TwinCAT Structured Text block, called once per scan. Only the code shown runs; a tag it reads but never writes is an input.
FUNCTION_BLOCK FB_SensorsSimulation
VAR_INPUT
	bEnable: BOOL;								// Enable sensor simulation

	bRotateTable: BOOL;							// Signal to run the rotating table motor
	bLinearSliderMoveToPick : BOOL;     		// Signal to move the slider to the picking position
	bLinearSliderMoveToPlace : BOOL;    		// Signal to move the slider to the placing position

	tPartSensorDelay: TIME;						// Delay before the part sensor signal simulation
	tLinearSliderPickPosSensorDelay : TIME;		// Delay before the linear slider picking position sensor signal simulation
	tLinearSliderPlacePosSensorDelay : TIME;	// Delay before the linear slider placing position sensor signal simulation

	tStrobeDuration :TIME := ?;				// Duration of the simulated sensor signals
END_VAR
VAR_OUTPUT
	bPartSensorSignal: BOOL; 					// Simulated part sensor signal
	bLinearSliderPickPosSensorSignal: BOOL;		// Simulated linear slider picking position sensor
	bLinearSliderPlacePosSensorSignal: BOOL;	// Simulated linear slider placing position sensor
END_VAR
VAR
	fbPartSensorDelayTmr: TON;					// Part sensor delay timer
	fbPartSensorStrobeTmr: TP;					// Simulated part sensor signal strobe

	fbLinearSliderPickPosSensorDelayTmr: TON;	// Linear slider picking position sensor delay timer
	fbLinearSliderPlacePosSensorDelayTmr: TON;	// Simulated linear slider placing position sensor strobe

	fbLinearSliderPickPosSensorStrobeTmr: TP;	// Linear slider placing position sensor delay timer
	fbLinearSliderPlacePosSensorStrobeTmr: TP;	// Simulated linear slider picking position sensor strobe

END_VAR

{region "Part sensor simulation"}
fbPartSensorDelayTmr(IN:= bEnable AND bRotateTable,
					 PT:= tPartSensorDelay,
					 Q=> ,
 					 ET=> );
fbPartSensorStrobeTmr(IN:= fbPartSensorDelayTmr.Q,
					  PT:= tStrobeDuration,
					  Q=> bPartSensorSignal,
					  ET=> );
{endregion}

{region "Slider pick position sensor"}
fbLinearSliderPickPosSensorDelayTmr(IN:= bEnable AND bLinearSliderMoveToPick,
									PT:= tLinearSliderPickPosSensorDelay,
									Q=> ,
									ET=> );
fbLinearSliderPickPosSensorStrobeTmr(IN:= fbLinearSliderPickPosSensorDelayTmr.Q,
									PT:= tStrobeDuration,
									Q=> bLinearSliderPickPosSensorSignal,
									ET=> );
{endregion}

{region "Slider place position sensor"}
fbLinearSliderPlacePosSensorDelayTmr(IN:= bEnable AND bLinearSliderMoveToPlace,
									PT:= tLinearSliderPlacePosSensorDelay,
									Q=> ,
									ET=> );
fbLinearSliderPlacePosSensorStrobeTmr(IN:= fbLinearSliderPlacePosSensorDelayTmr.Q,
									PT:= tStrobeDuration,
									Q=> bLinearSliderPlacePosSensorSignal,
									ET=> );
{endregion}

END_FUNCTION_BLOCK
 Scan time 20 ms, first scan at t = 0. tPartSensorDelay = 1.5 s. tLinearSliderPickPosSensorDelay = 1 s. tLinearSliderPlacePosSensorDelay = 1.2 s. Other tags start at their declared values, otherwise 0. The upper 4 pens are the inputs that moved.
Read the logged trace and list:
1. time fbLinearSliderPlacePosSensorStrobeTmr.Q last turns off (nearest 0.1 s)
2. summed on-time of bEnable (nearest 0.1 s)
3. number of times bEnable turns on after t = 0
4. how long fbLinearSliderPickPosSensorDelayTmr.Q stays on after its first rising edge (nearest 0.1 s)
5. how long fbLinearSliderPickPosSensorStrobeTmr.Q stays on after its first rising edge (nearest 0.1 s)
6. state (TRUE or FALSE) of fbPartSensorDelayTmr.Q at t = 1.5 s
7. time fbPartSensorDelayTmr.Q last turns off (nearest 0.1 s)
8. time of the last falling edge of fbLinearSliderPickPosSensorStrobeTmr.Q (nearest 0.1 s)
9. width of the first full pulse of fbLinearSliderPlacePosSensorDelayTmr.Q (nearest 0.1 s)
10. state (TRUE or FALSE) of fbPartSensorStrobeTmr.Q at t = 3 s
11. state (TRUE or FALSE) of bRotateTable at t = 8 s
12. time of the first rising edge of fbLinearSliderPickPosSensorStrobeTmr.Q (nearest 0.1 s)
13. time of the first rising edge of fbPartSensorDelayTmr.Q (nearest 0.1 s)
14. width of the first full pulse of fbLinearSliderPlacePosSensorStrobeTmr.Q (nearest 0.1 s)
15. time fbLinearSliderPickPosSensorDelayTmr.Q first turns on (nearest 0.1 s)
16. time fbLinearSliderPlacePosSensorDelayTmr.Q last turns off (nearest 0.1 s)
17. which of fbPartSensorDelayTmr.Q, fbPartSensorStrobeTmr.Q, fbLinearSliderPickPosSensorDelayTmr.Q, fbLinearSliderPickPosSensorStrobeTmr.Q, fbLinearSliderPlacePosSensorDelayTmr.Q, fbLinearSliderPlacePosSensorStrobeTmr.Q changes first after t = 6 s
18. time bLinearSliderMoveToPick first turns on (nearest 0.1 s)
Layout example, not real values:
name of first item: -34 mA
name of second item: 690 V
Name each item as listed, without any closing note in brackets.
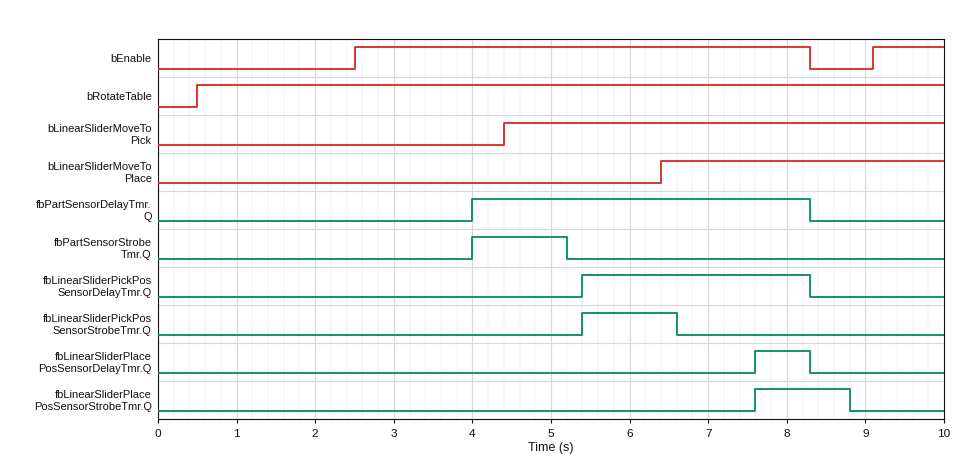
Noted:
time fbLinearSliderPlacePosSensorStrobeTmr.Q last turns off: 8.8 s
summed on-time of bEnable: 6.7 s
number of times bEnable turns on after t = 0: 2
how long fbLinearSliderPickPosSensorDelayTmr.Q stays on after its first rising edge: 2.9 s
how long fbLinearSliderPickPosSensorStrobeTmr.Q stays on after its first rising edge: 1.2 s
state (TRUE or FALSE) of fbPartSensorDelayTmr.Q at t = 1.5 s: FALSE
time fbPartSensorDelayTmr.Q last turns off: 8.3 s
time of the last falling edge of fbLinearSliderPickPosSensorStrobeTmr.Q: 6.6 s
width of the first full pulse of fbLinearSliderPlacePosSensorDelayTmr.Q: 0.7 s
state (TRUE or FALSE) of fbPartSensorStrobeTmr.Q at t = 3 s: FALSE
state (TRUE or FALSE) of bRotateTable at t = 8 s: TRUE
time of the first rising edge of fbLinearSliderPickPosSensorStrobeTmr.Q: 5.4 s
time of the first rising edge of fbPartSensorDelayTmr.Q: 4.0 s
width of the first full pulse of fbLinearSliderPlacePosSensorStrobeTmr.Q: 1.2 s
time fbLinearSliderPickPosSensorDelayTmr.Q first turns on: 5.4 s
time fbLinearSliderPlacePosSensorDelayTmr.Q last turns off: 8.3 s
which of fbPartSensorDelayTmr.Q, fbPartSensorStrobeTmr.Q, fbLinearSliderPickPosSensorDelayTmr.Q, fbLinearSliderPickPosSensorStrobeTmr.Q, fbLinearSliderPlacePosSensorDelayTmr.Q, fbLinearSliderPlacePosSensorStrobeTmr.Q changes first after t = 6 s: fbLinearSliderPickPosSensorStrobeTmr.Q
time bLinearSliderMoveToPick first turns on: 4.4 s
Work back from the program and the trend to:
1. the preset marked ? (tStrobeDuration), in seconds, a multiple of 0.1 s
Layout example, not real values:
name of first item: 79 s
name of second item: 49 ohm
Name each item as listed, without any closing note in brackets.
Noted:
the preset marked ? (tStrobeDuration), in seconds, a multiple of 0.1 s: 1.2 s
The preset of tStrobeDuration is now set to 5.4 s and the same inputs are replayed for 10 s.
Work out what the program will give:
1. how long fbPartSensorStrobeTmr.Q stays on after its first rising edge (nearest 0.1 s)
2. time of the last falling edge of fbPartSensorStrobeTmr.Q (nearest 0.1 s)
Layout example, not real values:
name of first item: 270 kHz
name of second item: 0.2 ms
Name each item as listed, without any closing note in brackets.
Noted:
how long fbPartSensorStrobeTmr.Q stays on after its first rising edge: 5.4 s
time of the last falling edge of fbPartSensorStrobeTmr.Q: 9.4 s
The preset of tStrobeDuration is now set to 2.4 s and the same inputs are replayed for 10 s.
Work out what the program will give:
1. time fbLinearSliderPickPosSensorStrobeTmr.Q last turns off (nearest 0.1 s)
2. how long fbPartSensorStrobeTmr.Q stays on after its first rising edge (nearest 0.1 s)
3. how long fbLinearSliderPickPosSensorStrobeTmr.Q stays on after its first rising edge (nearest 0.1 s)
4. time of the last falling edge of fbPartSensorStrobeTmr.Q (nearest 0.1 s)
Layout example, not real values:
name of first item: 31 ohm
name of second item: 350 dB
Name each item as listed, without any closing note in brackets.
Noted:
time fbLinearSliderPickPosSensorStrobeTmr.Q last turns off: 7.8 s
how long fbPartSensorStrobeTmr.Q stays on after its first rising edge: 2.4 s
how long fbLinearSliderPickPosSensorStrobeTmr.Q stays on after its first rising edge: 2.4 s
time of the last falling edge of fbPartSensorStrobeTmr.Q: 6.4 s
